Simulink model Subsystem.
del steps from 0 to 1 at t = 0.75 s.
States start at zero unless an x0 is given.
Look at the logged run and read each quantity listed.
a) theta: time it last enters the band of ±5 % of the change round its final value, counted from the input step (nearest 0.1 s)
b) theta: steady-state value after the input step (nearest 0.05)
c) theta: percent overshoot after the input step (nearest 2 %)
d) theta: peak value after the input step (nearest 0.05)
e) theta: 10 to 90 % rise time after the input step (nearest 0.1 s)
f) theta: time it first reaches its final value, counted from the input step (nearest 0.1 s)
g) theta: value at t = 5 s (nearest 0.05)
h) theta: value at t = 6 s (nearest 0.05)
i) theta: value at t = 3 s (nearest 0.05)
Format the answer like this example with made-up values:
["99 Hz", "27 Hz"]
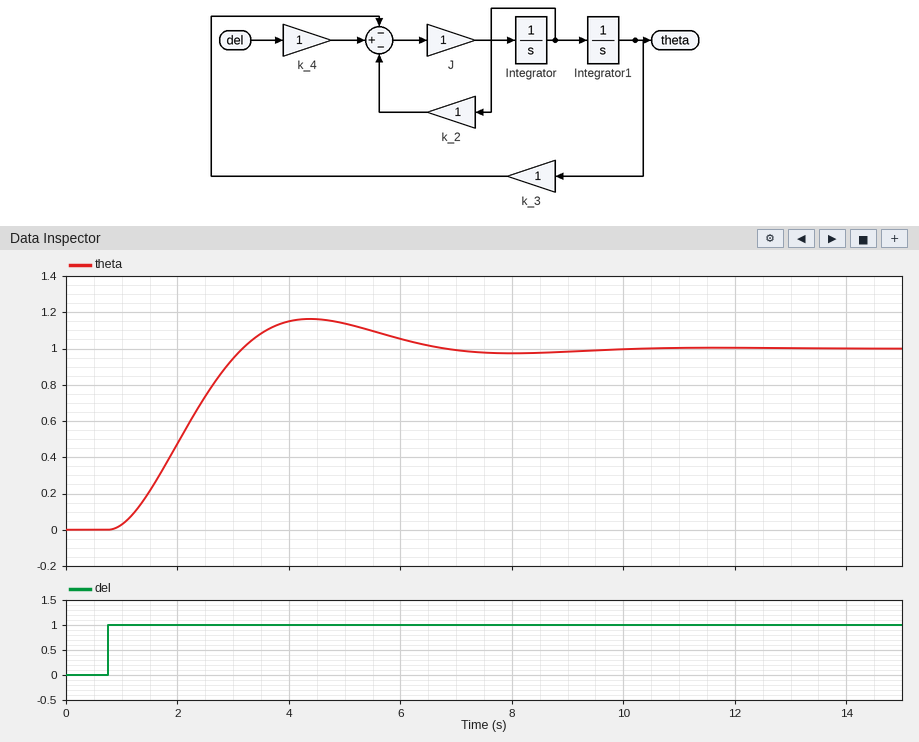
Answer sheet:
["5.3 s", "1.00", "16 %", "1.15", "1.6 s", "2.4 s", "1.15", "1.05", "0.95"]
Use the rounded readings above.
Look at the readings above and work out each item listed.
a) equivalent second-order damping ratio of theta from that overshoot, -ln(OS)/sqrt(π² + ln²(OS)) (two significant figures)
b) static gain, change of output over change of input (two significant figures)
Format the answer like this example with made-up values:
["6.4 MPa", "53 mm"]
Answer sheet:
["0.50", "1.0"]
